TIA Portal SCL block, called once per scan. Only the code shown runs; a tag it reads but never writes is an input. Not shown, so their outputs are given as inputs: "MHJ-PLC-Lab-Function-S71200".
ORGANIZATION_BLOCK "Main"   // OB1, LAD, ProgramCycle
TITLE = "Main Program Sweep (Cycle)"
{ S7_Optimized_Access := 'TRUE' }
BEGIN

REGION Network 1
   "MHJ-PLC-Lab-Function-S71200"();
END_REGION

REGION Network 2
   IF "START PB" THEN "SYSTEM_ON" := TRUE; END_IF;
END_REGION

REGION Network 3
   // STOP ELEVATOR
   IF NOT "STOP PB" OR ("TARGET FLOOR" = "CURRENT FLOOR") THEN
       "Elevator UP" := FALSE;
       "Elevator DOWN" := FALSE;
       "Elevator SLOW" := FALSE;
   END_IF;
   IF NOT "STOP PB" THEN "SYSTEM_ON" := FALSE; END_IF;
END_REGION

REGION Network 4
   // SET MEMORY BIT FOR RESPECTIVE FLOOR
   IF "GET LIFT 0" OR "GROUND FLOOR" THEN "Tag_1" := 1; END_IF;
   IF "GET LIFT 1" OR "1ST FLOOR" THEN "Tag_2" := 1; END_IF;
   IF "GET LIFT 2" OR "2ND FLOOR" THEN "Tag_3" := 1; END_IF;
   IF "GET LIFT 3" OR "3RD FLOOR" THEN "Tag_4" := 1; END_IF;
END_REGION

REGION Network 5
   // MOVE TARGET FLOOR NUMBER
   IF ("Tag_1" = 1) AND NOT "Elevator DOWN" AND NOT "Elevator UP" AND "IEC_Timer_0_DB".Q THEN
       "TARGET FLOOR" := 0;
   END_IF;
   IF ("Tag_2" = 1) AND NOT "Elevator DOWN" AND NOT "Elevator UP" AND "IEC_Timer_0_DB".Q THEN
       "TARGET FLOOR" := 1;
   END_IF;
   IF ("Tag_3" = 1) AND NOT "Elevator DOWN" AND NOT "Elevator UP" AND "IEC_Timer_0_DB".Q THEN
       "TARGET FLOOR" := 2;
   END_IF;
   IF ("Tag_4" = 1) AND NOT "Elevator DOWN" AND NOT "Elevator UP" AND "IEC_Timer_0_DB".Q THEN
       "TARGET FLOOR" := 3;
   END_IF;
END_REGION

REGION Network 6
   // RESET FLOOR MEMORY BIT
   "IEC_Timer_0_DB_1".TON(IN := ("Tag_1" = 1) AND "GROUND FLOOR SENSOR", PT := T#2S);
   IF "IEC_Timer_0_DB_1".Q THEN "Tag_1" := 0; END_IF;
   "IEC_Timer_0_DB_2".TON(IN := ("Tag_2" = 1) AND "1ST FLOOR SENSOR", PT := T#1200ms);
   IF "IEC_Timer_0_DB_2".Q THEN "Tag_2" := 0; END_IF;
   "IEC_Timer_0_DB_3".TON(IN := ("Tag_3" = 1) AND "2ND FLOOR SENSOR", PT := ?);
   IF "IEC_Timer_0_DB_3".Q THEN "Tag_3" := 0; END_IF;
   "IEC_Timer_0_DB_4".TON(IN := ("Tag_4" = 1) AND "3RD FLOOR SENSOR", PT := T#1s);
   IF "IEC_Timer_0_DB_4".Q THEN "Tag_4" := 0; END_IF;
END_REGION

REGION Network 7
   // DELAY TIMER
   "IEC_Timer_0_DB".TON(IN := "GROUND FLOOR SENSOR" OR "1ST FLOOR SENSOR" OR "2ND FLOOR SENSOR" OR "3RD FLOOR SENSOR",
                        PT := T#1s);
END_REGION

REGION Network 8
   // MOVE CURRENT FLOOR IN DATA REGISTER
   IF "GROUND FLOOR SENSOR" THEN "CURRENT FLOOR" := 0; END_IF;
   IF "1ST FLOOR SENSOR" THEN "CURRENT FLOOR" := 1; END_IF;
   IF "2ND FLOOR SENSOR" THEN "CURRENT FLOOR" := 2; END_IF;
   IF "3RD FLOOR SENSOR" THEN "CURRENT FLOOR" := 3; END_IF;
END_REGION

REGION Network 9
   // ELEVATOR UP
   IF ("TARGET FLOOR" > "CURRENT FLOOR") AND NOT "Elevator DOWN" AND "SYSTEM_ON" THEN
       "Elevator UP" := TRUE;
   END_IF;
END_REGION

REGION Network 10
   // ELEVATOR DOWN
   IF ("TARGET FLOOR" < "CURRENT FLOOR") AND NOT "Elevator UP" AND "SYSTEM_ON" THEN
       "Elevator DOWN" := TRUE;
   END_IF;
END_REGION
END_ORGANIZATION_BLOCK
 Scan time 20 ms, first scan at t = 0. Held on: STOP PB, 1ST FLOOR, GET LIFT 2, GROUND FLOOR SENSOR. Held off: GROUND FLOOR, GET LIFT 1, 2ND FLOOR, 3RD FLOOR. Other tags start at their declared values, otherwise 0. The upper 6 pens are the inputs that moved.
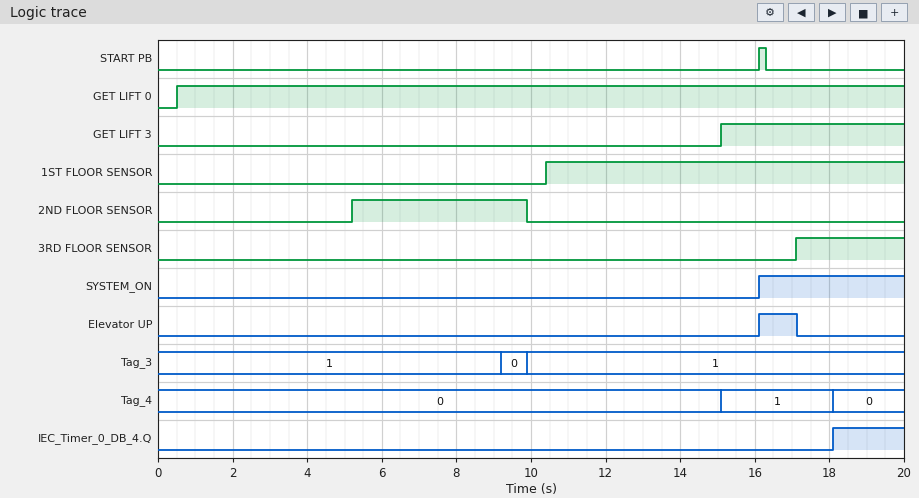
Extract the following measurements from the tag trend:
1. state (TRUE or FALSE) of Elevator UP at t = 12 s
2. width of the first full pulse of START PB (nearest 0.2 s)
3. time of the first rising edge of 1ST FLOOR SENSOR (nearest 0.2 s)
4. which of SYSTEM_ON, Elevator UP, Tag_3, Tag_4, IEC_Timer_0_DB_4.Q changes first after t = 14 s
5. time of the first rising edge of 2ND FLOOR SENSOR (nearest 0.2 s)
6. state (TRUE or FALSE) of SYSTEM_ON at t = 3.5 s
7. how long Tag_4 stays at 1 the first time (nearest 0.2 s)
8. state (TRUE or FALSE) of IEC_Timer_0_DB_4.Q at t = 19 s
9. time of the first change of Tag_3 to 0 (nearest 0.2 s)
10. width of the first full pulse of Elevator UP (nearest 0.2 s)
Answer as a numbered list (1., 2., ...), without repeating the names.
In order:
1. FALSE
2. 0.2 s
3. 10.4 s
4. Tag_4
5. 5.2 s
6. FALSE
7. 3.0 s
8. TRUE
9. 9.2 s
10. 1.0 s
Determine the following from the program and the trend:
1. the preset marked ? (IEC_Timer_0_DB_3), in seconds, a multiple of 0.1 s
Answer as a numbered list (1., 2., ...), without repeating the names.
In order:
1. 4.0 s
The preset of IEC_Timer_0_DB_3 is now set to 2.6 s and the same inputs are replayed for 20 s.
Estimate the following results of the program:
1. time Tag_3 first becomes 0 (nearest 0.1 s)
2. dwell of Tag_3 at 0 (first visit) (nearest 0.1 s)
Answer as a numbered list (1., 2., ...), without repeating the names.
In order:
1. 7.8 s
2. 2.1 s
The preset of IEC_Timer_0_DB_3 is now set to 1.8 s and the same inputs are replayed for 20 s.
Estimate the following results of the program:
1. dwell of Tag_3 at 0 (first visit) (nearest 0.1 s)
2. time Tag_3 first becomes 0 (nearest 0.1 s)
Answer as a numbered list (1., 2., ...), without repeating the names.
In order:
1. 2.9 s
2. 7.0 s
